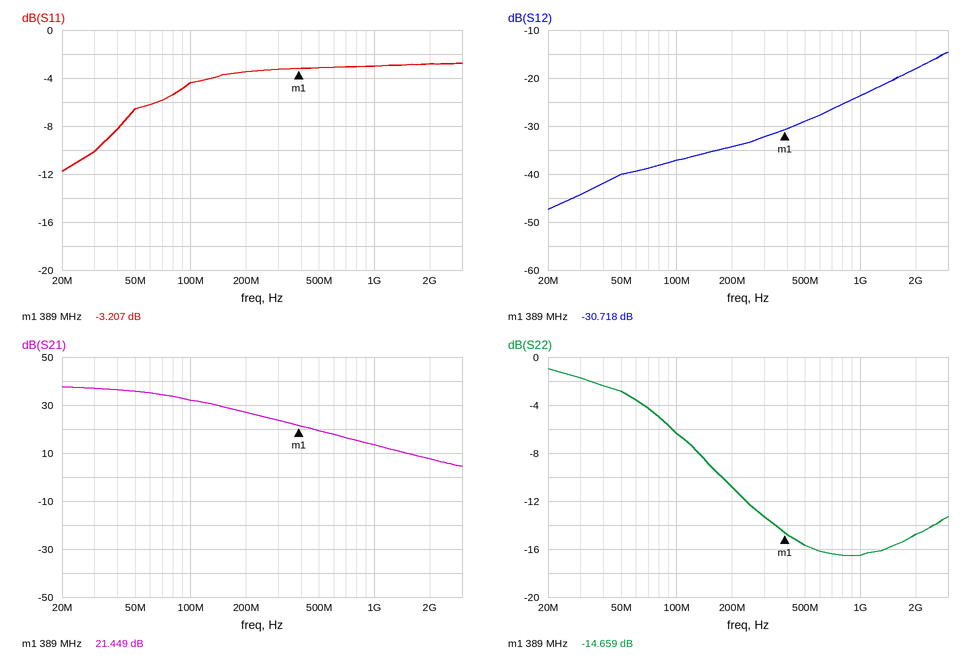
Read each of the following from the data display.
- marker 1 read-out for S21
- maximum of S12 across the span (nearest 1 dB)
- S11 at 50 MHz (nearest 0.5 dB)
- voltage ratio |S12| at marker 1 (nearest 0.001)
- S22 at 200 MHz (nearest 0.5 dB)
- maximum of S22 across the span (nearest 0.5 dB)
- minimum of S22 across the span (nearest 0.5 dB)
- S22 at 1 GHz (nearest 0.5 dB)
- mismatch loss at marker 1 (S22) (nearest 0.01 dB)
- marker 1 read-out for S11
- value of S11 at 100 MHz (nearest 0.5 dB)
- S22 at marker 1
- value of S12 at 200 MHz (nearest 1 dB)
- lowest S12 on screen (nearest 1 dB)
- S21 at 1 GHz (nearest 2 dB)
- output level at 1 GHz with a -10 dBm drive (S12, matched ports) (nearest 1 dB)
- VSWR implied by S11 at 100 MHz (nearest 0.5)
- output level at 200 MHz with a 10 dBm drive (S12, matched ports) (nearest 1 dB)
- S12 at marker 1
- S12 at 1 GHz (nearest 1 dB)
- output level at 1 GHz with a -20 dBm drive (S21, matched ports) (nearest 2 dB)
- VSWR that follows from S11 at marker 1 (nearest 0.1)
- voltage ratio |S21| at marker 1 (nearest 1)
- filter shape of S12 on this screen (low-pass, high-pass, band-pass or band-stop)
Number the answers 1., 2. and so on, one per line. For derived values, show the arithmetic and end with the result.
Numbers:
1. 21.449 dB
2. -15 dB
3. -6.5 dB
4. 10^(-30.718/20) ≈ 0.029
5. -11.0 dB
6. -1.0 dB
7. -16.5 dB
8. -16.5 dB
9. −10 log10(1 − 10^(-14.659/10)) ≈ 0.15 dB
10. -3.207 dB
11. -4.5 dB
12. -14.659 dB
13. -34 dB
14. -47 dB
15. 14 dB
16. -10 dBm + (-24 dB) = -34 dBm
17. |Γ| = 10^(-4.5/20) = 0.5957; VSWR = (1 + 0.5957)/(1 − 0.5957) ≈ 4.0
18. 10 dBm + (-34 dB) = -24 dBm
19. -30.718 dB
20. -24 dB
21. -20 dBm + (14 dB) = -6 dBm
22. (1 + 0.6913)/(1 − 0.6913) ≈ 5.5
23. 10^(21.449/20) ≈ 12
24. high-pass
